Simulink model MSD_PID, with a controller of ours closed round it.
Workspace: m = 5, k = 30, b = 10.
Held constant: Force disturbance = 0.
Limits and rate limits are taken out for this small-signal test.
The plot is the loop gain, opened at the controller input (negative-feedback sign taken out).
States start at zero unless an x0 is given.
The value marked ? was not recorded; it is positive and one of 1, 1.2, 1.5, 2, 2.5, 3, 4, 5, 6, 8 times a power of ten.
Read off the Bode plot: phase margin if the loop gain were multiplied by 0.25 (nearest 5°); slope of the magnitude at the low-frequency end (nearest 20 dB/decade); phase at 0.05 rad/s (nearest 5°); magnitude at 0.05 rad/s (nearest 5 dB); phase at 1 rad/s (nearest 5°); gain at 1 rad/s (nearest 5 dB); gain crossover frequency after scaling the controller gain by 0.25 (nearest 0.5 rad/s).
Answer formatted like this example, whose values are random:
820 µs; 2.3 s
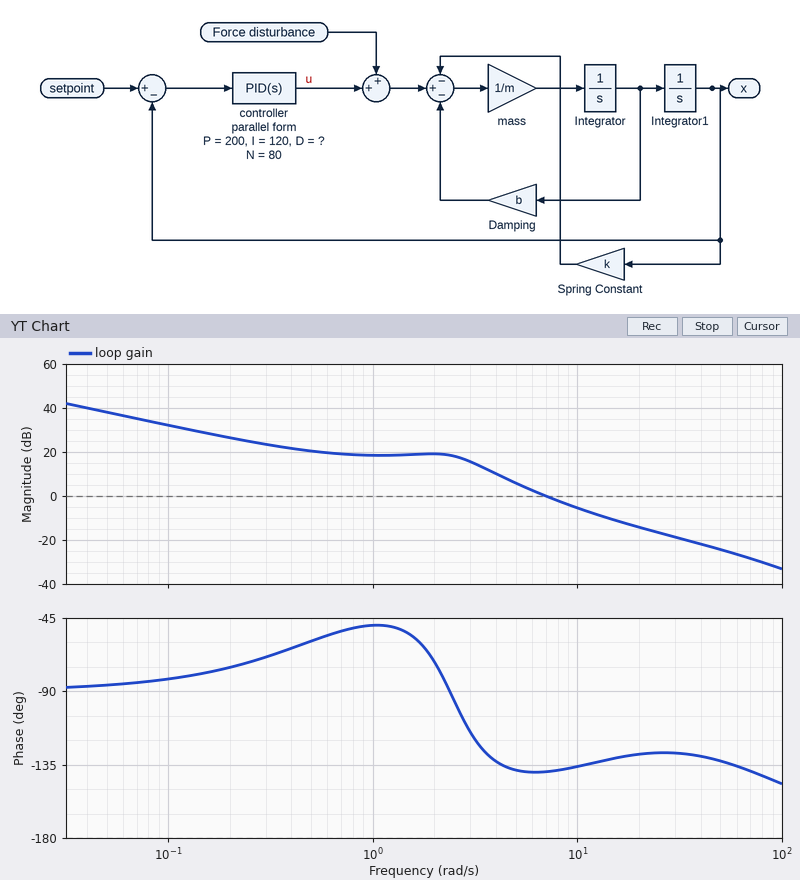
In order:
50°; -20 dB/decade; -85°; 40 dB; -50°; 20 dB; 3.5 rad/s
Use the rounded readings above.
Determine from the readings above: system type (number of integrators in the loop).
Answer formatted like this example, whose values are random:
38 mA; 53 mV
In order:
1
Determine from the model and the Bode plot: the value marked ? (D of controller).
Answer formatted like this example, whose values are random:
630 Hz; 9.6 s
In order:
15
